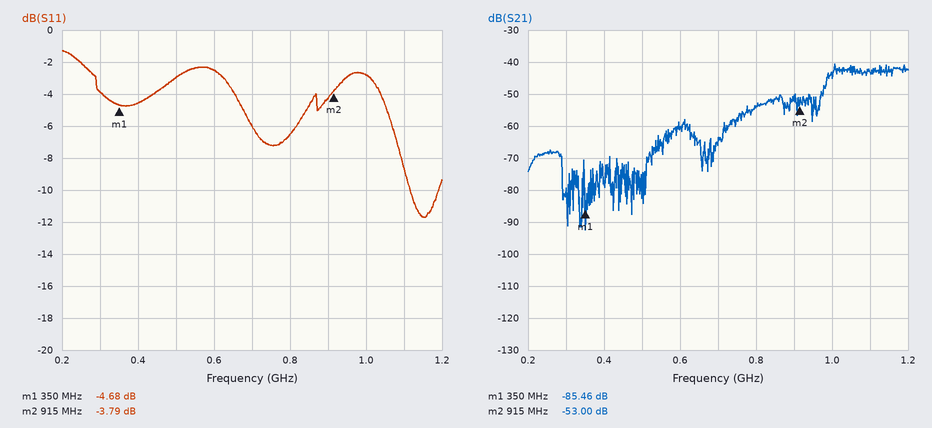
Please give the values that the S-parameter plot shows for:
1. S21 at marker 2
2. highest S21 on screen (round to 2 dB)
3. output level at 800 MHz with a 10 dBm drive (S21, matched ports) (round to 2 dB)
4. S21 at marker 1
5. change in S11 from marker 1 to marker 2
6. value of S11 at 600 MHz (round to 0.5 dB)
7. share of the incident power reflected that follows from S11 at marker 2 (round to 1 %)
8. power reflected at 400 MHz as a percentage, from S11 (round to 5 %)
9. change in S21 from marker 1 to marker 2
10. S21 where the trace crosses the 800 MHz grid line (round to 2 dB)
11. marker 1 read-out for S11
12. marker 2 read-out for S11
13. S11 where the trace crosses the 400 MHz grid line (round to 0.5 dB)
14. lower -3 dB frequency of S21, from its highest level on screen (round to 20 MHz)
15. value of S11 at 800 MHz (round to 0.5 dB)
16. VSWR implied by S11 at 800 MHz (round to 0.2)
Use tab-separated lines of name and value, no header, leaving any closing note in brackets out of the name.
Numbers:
S21 at marker 2	-53.00 dB
highest S21 on screen	-40 dB
output level at 800 MHz with a 10 dBm drive (S21, matched ports)	-44 dBm
S21 at marker 1	-85.46 dB
change in S11 from marker 1 to marker 2	0.89 dB
value of S11 at 600 MHz	-2.5 dB
share of the incident power reflected that follows from S11 at marker 2	42 %
power reflected at 400 MHz as a percentage, from S11	35 %
change in S21 from marker 1 to marker 2	32.46 dB
S21 where the trace crosses the 800 MHz grid line	-54 dB
marker 1 read-out for S11	-4.68 dB
marker 2 read-out for S11	-3.79 dB
S11 where the trace crosses the 400 MHz grid line	-4.5 dB
lower -3 dB frequency of S21, from its highest level on screen	1.00 GHz
value of S11 at 800 MHz	-6.5 dB
VSWR implied by S11 at 800 MHz	2.8
